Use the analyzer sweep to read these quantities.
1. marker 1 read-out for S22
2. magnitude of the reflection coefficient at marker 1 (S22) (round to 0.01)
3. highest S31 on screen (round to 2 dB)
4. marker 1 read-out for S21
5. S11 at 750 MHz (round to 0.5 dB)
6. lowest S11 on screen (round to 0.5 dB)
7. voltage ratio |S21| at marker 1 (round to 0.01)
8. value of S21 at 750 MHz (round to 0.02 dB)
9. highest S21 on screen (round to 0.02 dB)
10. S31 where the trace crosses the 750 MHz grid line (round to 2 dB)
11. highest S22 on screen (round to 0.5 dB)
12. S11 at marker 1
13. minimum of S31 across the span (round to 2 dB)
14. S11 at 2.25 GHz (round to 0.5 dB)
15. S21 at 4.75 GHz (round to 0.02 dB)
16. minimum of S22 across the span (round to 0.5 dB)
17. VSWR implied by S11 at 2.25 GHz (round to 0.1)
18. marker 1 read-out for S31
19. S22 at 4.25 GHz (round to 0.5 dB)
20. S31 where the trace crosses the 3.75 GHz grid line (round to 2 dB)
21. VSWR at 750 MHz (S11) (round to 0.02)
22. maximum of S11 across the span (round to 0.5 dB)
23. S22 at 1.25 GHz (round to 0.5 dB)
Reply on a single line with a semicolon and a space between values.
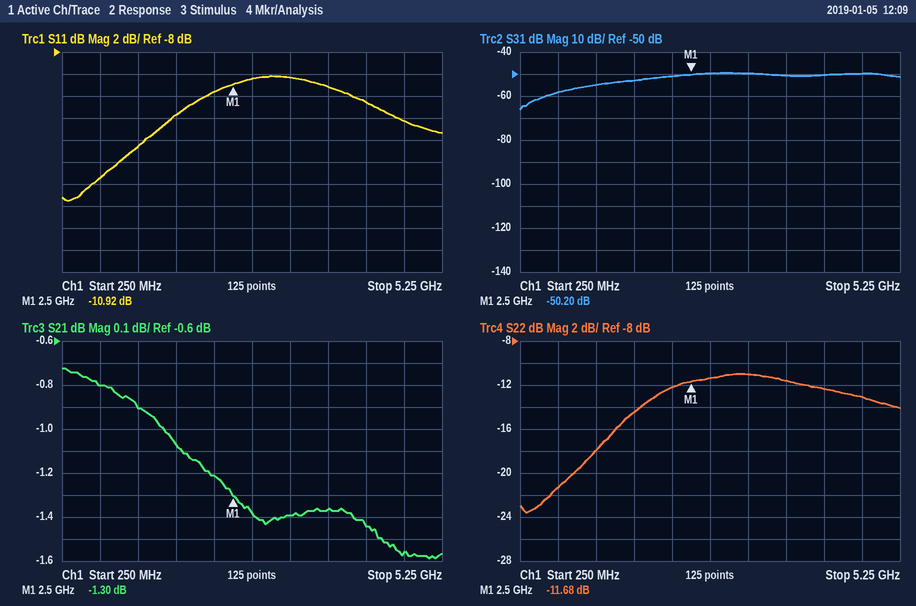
-11.68 dB; 0.26; -50 dB; -1.30 dB; -19.5 dB; -21.5 dB; 0.86; -0.80 dB; -0.72 dB; -58 dB; -11.0 dB; -10.92 dB; -66 dB; -11.5 dB; -1.56 dB; -23.5 dB; 1.7; -50.20 dB; -12.5 dB; -50 dB; 1.24; -10.0 dB; -18.0 dB
